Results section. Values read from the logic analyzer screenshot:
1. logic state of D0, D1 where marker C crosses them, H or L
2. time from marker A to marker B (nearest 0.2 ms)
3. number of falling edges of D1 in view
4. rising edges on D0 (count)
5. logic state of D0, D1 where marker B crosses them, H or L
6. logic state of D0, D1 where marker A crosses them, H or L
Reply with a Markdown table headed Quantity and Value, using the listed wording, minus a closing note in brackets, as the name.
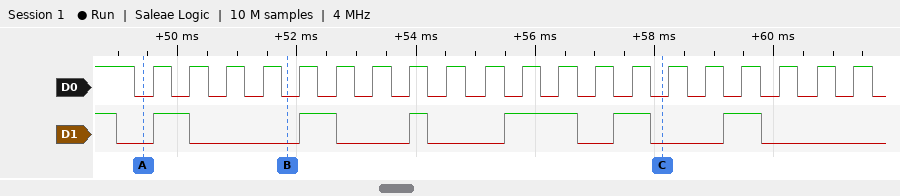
| Quantity | Value |
|---|---|
| logic state of D0, D1 where marker C crosses them, H or L | D0=L, D1=L |
| time from marker A to marker B | 2.4 ms |
| number of falling edges of D1 in view | 7 |
| rising edges on D0 | 20 |
| logic state of D0, D1 where marker B crosses them, H or L | D0=L, D1=L |
| logic state of D0, D1 where marker A crosses them, H or L | D0=L, D1=L |
